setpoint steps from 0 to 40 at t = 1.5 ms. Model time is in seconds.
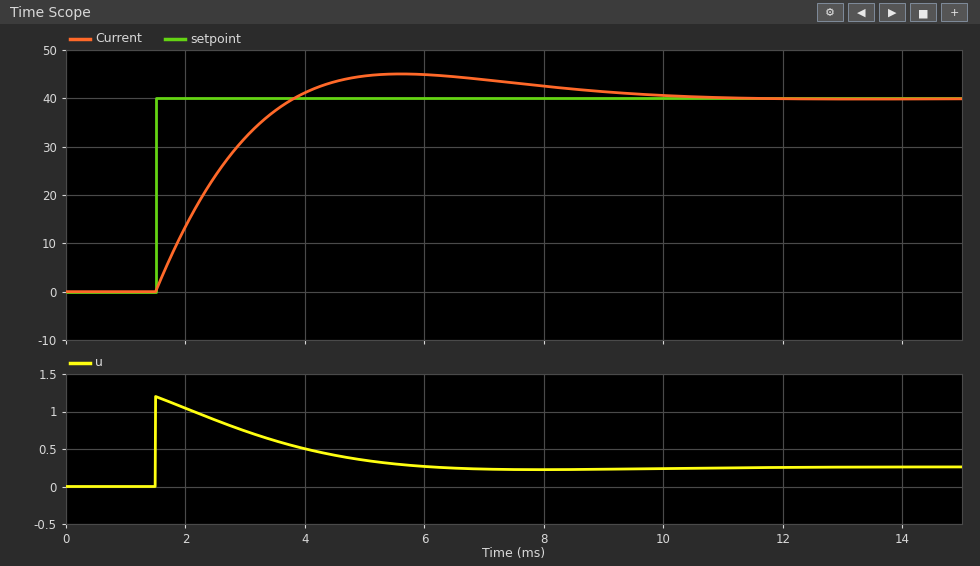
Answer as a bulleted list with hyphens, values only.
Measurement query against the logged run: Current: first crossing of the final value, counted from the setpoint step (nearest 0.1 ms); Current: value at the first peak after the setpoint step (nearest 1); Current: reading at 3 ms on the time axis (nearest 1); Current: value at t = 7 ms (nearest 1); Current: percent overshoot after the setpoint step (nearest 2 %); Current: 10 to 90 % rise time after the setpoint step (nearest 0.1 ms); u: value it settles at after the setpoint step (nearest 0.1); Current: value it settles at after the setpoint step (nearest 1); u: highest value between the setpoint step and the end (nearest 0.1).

- 2.3 ms
- 45
- 32
- 44
- 12 %
- 1.7 ms
- 0.3
- 40
- 1.2
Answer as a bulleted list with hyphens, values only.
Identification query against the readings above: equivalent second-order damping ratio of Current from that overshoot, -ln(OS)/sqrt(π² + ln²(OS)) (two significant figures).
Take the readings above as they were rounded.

- 0.56
